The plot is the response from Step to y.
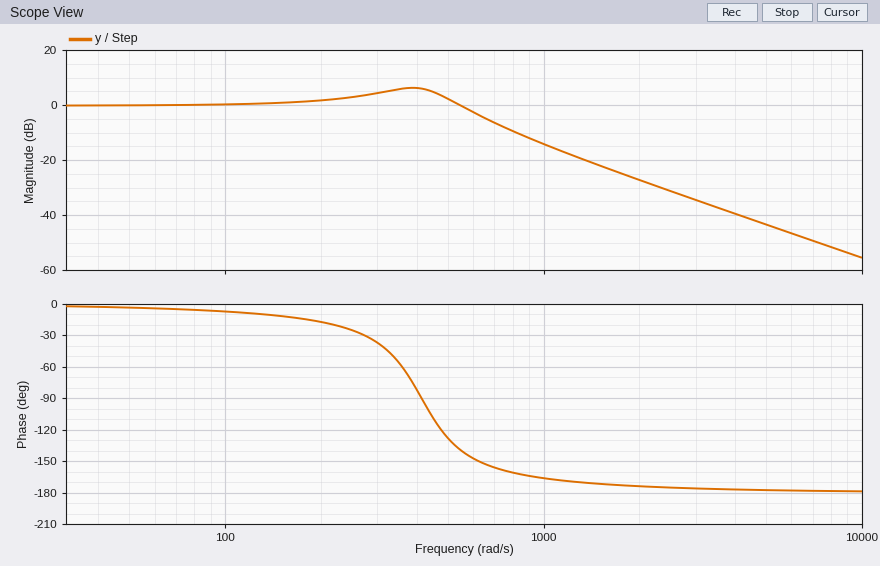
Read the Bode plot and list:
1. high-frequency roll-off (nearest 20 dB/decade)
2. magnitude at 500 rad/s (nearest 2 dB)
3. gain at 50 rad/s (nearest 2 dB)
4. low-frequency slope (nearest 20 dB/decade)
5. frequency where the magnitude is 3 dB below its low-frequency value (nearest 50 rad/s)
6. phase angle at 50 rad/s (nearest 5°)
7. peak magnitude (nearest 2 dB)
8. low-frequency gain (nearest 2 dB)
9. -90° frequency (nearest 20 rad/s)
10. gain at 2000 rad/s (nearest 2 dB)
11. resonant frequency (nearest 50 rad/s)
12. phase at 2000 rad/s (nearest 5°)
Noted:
-40 dB/decade
2 dB
0 dB
0 dB/decade
600 rad/s
-5°
6 dB
0 dB
420 rad/s
-28 dB
400 rad/s
-175°
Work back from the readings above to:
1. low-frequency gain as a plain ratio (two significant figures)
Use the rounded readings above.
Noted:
1.0
